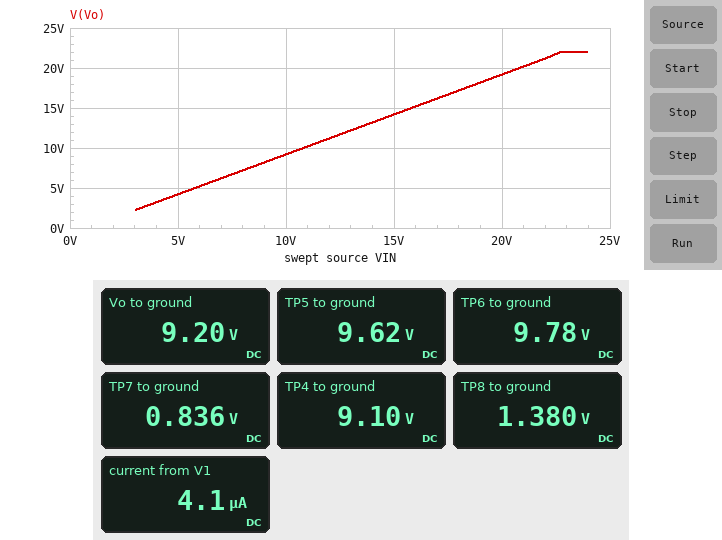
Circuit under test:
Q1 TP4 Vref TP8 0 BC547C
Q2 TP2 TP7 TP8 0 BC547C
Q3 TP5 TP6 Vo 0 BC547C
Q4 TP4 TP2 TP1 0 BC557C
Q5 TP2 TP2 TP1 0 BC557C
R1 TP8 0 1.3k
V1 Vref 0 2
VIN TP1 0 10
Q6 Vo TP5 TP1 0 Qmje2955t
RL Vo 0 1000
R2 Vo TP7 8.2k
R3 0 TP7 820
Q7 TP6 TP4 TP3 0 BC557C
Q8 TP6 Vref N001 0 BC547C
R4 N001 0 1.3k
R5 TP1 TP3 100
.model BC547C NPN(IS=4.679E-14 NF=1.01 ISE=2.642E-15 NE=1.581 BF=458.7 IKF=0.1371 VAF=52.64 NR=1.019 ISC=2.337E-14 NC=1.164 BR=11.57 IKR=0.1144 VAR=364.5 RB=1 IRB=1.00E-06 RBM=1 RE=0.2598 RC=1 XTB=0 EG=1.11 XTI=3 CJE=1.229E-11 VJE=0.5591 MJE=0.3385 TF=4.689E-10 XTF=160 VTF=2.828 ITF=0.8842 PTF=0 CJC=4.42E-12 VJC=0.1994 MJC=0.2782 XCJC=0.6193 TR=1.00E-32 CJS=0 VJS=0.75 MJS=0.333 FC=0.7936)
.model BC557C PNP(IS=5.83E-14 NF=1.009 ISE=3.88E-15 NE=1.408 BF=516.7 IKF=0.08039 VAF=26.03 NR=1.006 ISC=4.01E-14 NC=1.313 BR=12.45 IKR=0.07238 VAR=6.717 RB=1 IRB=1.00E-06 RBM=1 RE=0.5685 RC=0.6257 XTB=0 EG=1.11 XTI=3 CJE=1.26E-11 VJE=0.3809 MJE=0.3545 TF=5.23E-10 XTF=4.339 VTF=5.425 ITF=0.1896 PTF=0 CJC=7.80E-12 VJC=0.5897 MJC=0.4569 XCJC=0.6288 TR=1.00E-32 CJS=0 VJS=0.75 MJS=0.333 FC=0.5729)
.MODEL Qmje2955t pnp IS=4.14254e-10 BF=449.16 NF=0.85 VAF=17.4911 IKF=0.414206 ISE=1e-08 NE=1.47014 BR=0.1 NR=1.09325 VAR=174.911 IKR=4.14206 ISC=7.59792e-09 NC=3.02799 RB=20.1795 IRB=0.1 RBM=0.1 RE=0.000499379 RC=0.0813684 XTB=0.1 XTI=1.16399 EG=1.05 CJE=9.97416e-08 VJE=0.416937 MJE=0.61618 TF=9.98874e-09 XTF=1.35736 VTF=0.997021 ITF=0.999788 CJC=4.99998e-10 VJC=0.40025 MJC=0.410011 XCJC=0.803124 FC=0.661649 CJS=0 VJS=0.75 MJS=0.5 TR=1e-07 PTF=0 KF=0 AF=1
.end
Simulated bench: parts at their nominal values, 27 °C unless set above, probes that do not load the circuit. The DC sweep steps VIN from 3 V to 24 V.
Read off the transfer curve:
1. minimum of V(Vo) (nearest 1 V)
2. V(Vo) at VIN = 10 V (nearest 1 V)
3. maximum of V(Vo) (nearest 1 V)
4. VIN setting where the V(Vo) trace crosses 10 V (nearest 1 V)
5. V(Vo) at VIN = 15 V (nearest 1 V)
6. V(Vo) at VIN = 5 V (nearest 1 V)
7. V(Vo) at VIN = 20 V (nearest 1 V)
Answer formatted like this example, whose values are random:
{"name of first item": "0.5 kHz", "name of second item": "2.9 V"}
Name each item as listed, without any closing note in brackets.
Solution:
{"minimum of V(Vo)": "2 V", "V(Vo) at VIN = 10 V": "9 V", "maximum of V(Vo)": "22 V", "VIN setting where the V(Vo) trace crosses 10 V": "11 V", "V(Vo) at VIN = 15 V": "14 V", "V(Vo) at VIN = 5 V": "4 V", "V(Vo) at VIN = 20 V": "19 V"}
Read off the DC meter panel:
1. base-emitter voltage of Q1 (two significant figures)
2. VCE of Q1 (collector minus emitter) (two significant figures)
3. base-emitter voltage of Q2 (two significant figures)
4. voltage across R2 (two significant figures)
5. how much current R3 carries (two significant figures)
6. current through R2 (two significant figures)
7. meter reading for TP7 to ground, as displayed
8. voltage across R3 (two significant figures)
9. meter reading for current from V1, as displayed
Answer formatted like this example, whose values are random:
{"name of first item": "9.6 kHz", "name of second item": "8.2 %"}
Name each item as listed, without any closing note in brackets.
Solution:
{"base-emitter voltage of Q1": "620 mV", "VCE of Q1 (collector minus emitter)": "7.7 V", "base-emitter voltage of Q2": "-540 mV", "voltage across R2": "8.4 V", "how much current R3 carries": "1.0 mA", "current through R2": "1.0 mA", "meter reading for TP7 to ground, as displayed": "0.836 V", "voltage across R3": "840 mV", "meter reading for current from V1, as displayed": "4.1 µA"}
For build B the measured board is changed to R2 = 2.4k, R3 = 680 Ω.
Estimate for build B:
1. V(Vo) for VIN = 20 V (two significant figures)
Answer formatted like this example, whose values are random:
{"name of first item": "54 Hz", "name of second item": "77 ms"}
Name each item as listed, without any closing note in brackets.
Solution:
{"V(Vo) for VIN = 20 V": "9.1 V"}
